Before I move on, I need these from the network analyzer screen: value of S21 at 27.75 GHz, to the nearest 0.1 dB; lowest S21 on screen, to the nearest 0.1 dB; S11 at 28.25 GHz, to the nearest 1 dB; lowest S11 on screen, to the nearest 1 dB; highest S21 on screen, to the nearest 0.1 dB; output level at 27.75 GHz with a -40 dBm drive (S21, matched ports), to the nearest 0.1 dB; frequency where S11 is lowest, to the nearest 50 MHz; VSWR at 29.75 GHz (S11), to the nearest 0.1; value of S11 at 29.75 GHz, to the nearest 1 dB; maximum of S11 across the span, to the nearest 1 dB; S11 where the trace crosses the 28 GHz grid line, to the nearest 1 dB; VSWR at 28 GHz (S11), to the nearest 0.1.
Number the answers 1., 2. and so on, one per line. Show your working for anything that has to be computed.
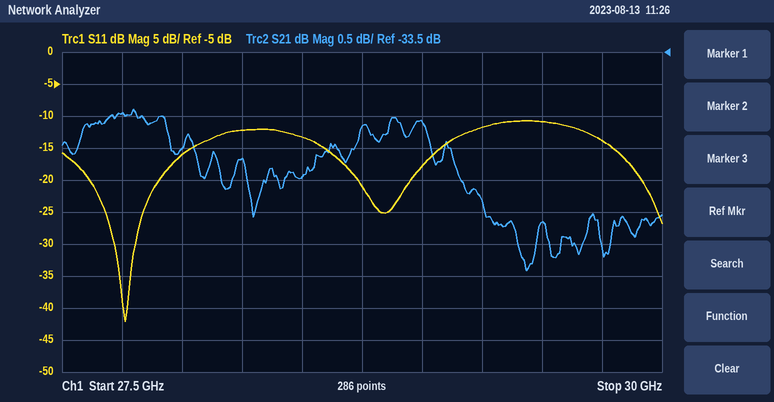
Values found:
1. -34.5 dB
2. -36.9 dB
3. -12 dB
4. -42 dB
5. -34.4 dB
6. -40 dBm + (-34.5 dB) = -74.5 dBm
7. 27.75 GHz
8. |Γ| = 10^(-14/20) = 0.1995; VSWR = (1 + 0.1995)/(1 − 0.1995) ≈ 1.5
9. -14 dB
10. -11 dB
11. -16 dB
12. |Γ| = 10^(-16/20) = 0.1585; VSWR = (1 + 0.1585)/(1 − 0.1585) ≈ 1.4
